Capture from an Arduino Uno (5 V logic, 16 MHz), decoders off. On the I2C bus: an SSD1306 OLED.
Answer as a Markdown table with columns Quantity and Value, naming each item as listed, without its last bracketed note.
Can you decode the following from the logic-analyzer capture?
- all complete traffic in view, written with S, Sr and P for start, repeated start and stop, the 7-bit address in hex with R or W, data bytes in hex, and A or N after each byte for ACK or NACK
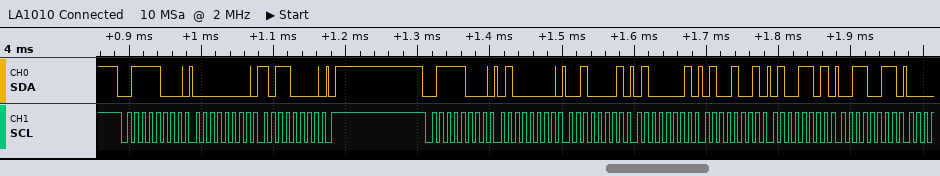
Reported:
| Quantity | Value |
|---|---|
| all complete traffic in view, written with S, Sr and P for start, repeated start and stop, the 7-bit address in hex with R or W, data bytes in hex, and A or N after each byte for ACK or NACK | S 3CW A 00 A B0 A P S 3CW A 40 A 21 A 41 A 49 A 4D A 33 A |
